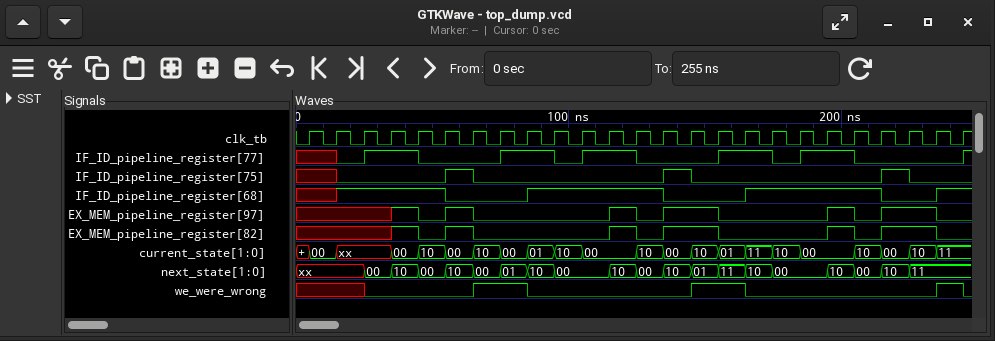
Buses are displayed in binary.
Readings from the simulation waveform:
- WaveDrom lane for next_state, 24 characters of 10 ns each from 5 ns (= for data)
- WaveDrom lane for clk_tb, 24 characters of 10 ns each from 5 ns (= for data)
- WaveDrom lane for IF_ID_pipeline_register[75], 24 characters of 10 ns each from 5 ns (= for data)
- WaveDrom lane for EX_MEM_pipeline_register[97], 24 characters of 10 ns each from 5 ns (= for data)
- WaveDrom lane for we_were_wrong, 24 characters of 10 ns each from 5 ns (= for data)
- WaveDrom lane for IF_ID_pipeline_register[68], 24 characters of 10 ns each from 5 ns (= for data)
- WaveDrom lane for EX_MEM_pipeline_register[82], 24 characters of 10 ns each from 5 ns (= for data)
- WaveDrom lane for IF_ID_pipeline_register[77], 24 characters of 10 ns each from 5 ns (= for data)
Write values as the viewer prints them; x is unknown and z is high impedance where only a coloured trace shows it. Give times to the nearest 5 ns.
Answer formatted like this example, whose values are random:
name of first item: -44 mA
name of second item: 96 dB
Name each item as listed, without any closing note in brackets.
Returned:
WaveDrom lane for next_state, 24 characters of 10 ns each from 5 ns: {name: 'next_state', wave: 'x.========.=======.====.', data: '00 10 00 10 00 01 10 00 10 00 10 01 11 10 00 10 00 10 11'}
WaveDrom lane for clk_tb, 24 characters of 10 ns each from 5 ns: {name: 'clk_tb', wave: 'p.......................'}
WaveDrom lane for IF_ID_pipeline_register[75], 24 characters of 10 ns each from 5 ns: {name: 'IF_ID_pipeline_register[75]', wave: 'x0...10......10......10.'}
WaveDrom lane for EX_MEM_pipeline_register[97], 24 characters of 10 ns each from 5 ns: {name: 'EX_MEM_pipeline_register[97]', wave: 'x..1010....101.0...101.0'}
WaveDrom lane for we_were_wrong, 24 characters of 10 ns each from 5 ns: {name: 'we_were_wrong', wave: 'x.0...1.0.....1.0......1'}
WaveDrom lane for IF_ID_pipeline_register[68], 24 characters of 10 ns each from 5 ns: {name: 'IF_ID_pipeline_register[68]', wave: 'x1...0..1....0..1....0.1'}
WaveDrom lane for EX_MEM_pipeline_register[82], 24 characters of 10 ns each from 5 ns: {name: 'EX_MEM_pipeline_register[82]', wave: 'x..1010....101.0...101.0'}
WaveDrom lane for IF_ID_pipeline_register[77], 24 characters of 10 ns each from 5 ns: {name: 'IF_ID_pipeline_register[77]', wave: 'x01.0..1.01.0..1.01.0...'}
